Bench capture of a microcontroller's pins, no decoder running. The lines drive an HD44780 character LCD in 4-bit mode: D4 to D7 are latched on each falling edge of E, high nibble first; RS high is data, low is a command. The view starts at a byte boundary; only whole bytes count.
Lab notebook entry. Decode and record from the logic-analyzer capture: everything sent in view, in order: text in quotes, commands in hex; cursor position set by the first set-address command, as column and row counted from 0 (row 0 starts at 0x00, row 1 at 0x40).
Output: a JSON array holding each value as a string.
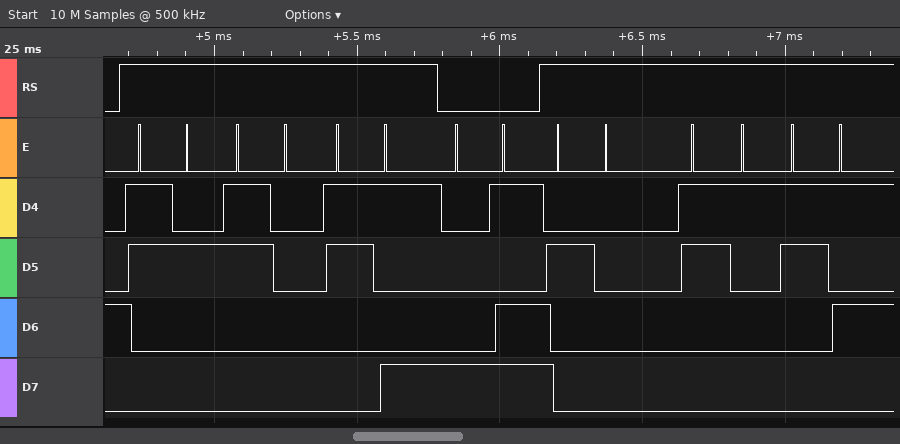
["\"209\" 0x8D \" 15\"", "column 13, row 0"]
